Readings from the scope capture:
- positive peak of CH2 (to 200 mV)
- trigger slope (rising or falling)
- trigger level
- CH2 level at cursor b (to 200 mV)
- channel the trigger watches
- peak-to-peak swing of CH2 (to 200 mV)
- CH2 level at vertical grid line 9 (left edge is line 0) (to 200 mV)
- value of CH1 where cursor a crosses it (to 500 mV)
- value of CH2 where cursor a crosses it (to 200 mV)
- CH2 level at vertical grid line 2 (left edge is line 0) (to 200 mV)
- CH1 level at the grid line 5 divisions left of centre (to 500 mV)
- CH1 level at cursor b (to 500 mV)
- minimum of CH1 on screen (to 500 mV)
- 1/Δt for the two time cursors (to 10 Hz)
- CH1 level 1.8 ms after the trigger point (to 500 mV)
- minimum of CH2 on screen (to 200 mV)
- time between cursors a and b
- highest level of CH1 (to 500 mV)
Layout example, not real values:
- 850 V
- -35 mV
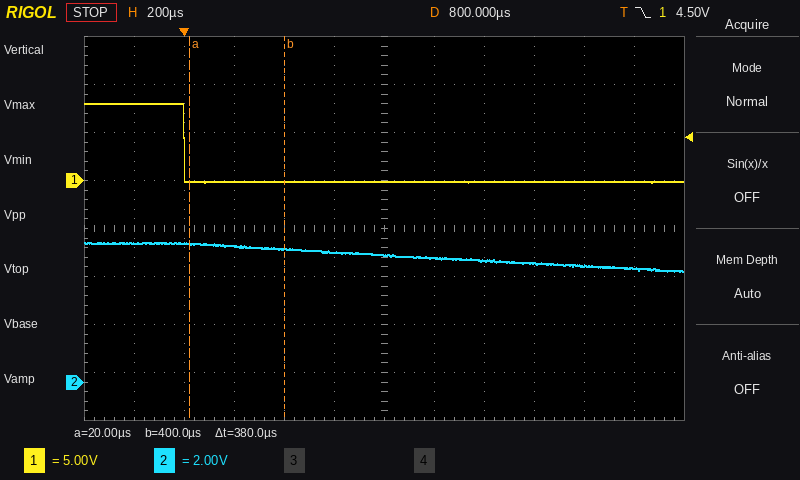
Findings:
- 5.8 V
- falling
- 4.50 V
- 5.6 V
- CH1
- 1.2 V
- 5.0 V
- 0.0 V
- 5.8 V
- 5.8 V
- 8.0 V
- 0.0 V
- 0.0 V
- 2.63 kHz
- 0.0 V
- 4.6 V
- 380 µs
- 8.0 V
